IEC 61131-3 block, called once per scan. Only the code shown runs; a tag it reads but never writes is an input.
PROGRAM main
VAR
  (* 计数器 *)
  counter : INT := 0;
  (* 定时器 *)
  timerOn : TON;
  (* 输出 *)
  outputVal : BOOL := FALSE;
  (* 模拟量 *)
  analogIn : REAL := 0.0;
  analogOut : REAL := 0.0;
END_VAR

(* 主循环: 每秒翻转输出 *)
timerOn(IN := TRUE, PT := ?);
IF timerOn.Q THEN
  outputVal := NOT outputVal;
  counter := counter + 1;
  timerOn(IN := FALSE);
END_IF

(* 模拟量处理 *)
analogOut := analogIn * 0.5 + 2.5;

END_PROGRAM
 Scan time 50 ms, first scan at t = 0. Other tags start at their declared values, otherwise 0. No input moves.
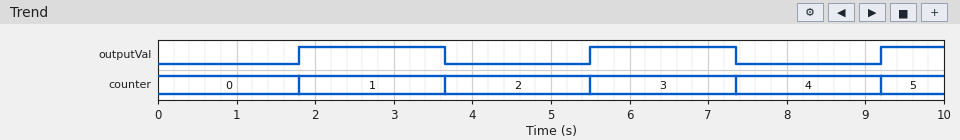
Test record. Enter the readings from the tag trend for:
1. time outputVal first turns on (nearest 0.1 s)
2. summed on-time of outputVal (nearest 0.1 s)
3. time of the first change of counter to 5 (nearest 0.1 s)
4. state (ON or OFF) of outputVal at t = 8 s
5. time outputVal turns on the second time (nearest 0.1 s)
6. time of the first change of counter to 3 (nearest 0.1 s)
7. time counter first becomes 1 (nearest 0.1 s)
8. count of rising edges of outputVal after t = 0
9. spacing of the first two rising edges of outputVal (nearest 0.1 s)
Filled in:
1.8 s
4.5 s
9.2 s
OFF
5.5 s
5.5 s
1.8 s
3
3.7 s
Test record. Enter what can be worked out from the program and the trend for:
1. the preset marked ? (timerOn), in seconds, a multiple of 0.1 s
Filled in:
1.8 s
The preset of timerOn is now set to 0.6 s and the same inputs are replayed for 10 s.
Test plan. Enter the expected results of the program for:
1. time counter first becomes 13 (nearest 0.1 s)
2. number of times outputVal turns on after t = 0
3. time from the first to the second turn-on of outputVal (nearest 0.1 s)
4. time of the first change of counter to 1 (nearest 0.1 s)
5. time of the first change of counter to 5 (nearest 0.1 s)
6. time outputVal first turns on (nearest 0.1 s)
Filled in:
8.4 s
8
1.3 s
0.6 s
3.2 s
0.6 s
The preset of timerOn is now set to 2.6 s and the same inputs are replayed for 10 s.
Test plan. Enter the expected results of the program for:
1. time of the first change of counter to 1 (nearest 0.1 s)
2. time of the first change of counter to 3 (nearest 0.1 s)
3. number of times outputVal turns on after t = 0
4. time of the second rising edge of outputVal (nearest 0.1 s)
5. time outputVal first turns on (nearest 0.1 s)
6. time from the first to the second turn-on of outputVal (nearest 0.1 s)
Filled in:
2.6 s
7.9 s
2
7.9 s
2.6 s
5.3 s
